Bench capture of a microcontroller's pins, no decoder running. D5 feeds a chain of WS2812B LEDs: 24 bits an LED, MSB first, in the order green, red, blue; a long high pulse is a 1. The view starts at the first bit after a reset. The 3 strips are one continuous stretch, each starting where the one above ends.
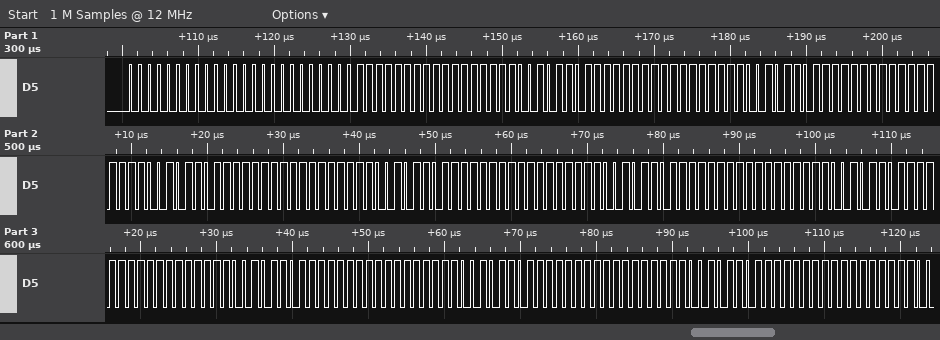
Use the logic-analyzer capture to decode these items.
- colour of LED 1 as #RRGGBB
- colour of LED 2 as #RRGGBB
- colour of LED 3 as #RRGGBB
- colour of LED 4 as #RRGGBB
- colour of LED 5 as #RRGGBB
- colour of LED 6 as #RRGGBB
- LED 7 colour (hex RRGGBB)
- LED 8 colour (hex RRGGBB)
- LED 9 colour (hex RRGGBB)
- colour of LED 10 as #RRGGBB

#000000
#FFFF96
#FFFF96
#FFFF96
#FFFF96
#FFFF96
#FFFF96
#FFFF96
#FFFF96
#FFFF96
